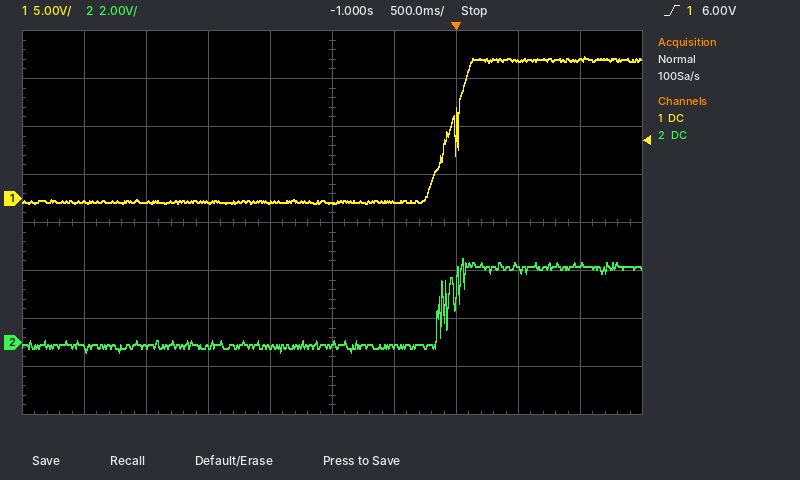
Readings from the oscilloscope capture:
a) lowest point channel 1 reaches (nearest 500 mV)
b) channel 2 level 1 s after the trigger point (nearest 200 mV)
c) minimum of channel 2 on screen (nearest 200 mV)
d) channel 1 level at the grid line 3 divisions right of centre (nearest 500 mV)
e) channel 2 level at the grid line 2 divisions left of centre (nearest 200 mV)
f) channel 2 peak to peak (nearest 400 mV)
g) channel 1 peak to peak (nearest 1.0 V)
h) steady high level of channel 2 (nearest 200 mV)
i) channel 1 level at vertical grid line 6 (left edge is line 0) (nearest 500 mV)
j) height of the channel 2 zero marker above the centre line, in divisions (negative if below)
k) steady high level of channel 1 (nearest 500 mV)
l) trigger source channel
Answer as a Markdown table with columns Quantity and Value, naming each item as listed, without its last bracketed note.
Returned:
| Quantity | Value |
|---|---|
| lowest point channel 1 reaches | -500 mV |
| channel 2 level 1 s after the trigger point | 3.2 V |
| minimum of channel 2 on screen | -400 mV |
| channel 1 level at the grid line 3 divisions right of centre | 14.5 V |
| channel 2 level at the grid line 2 divisions left of centre | -200 mV |
| channel 2 peak to peak | 4.0 V |
| channel 1 peak to peak | 15.0 V |
| steady high level of channel 2 | 3.2 V |
| channel 1 level at vertical grid line 6 (left edge is line 0) | -500 mV |
| height of the channel 2 zero marker above the centre line, in divisions | -2.5 div |
| steady high level of channel 1 | 14.5 V |
| trigger source channel | channel 1 |
